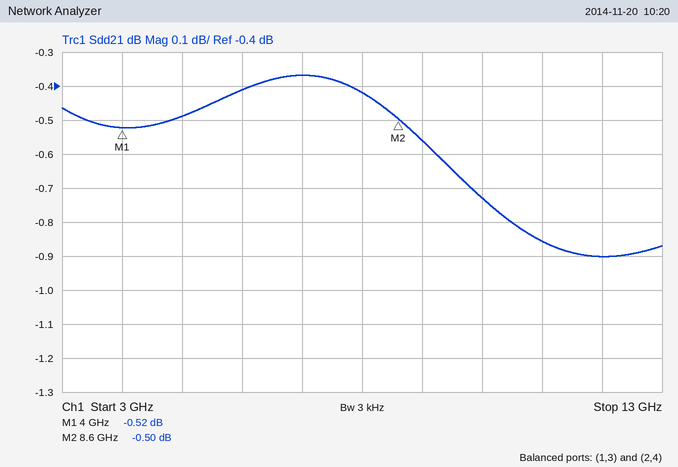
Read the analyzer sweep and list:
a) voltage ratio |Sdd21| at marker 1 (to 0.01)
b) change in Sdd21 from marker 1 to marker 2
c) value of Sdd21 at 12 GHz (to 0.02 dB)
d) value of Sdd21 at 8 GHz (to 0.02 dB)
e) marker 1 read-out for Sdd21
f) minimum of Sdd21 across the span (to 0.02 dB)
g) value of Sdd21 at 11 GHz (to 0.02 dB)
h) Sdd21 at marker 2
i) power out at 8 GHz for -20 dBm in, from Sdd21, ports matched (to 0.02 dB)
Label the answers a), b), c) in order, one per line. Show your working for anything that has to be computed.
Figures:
a) 10^(-0.52/20) ≈ 0.94
b) -0.5 − (-0.52) = 0.02 dB
c) -0.90 dB
d) -0.42 dB
e) -0.52 dB
f) -0.90 dB
g) -0.86 dB
h) -0.50 dB
i) -20 dBm + (-0.42 dB) = -20.42 dBm
